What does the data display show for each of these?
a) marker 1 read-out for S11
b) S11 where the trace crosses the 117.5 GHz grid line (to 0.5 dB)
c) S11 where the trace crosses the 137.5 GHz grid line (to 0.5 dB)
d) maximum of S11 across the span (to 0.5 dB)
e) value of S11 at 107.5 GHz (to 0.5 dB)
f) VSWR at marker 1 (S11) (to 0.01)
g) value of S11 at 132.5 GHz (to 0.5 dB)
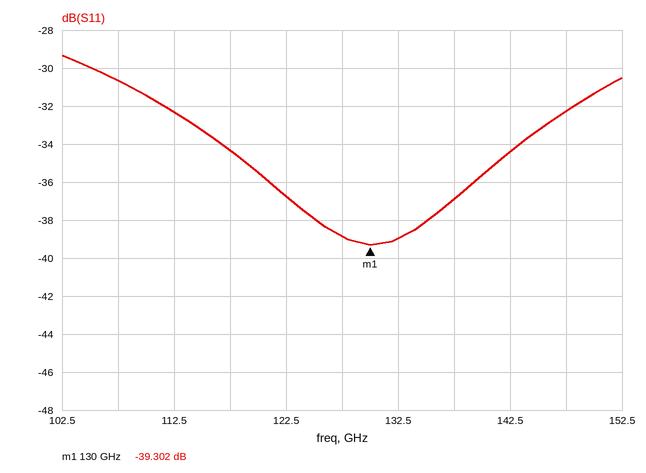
-39.302 dB
-34.5 dB
-37.0 dB
-29.5 dB
-30.5 dB
1.02
-39.0 dB
